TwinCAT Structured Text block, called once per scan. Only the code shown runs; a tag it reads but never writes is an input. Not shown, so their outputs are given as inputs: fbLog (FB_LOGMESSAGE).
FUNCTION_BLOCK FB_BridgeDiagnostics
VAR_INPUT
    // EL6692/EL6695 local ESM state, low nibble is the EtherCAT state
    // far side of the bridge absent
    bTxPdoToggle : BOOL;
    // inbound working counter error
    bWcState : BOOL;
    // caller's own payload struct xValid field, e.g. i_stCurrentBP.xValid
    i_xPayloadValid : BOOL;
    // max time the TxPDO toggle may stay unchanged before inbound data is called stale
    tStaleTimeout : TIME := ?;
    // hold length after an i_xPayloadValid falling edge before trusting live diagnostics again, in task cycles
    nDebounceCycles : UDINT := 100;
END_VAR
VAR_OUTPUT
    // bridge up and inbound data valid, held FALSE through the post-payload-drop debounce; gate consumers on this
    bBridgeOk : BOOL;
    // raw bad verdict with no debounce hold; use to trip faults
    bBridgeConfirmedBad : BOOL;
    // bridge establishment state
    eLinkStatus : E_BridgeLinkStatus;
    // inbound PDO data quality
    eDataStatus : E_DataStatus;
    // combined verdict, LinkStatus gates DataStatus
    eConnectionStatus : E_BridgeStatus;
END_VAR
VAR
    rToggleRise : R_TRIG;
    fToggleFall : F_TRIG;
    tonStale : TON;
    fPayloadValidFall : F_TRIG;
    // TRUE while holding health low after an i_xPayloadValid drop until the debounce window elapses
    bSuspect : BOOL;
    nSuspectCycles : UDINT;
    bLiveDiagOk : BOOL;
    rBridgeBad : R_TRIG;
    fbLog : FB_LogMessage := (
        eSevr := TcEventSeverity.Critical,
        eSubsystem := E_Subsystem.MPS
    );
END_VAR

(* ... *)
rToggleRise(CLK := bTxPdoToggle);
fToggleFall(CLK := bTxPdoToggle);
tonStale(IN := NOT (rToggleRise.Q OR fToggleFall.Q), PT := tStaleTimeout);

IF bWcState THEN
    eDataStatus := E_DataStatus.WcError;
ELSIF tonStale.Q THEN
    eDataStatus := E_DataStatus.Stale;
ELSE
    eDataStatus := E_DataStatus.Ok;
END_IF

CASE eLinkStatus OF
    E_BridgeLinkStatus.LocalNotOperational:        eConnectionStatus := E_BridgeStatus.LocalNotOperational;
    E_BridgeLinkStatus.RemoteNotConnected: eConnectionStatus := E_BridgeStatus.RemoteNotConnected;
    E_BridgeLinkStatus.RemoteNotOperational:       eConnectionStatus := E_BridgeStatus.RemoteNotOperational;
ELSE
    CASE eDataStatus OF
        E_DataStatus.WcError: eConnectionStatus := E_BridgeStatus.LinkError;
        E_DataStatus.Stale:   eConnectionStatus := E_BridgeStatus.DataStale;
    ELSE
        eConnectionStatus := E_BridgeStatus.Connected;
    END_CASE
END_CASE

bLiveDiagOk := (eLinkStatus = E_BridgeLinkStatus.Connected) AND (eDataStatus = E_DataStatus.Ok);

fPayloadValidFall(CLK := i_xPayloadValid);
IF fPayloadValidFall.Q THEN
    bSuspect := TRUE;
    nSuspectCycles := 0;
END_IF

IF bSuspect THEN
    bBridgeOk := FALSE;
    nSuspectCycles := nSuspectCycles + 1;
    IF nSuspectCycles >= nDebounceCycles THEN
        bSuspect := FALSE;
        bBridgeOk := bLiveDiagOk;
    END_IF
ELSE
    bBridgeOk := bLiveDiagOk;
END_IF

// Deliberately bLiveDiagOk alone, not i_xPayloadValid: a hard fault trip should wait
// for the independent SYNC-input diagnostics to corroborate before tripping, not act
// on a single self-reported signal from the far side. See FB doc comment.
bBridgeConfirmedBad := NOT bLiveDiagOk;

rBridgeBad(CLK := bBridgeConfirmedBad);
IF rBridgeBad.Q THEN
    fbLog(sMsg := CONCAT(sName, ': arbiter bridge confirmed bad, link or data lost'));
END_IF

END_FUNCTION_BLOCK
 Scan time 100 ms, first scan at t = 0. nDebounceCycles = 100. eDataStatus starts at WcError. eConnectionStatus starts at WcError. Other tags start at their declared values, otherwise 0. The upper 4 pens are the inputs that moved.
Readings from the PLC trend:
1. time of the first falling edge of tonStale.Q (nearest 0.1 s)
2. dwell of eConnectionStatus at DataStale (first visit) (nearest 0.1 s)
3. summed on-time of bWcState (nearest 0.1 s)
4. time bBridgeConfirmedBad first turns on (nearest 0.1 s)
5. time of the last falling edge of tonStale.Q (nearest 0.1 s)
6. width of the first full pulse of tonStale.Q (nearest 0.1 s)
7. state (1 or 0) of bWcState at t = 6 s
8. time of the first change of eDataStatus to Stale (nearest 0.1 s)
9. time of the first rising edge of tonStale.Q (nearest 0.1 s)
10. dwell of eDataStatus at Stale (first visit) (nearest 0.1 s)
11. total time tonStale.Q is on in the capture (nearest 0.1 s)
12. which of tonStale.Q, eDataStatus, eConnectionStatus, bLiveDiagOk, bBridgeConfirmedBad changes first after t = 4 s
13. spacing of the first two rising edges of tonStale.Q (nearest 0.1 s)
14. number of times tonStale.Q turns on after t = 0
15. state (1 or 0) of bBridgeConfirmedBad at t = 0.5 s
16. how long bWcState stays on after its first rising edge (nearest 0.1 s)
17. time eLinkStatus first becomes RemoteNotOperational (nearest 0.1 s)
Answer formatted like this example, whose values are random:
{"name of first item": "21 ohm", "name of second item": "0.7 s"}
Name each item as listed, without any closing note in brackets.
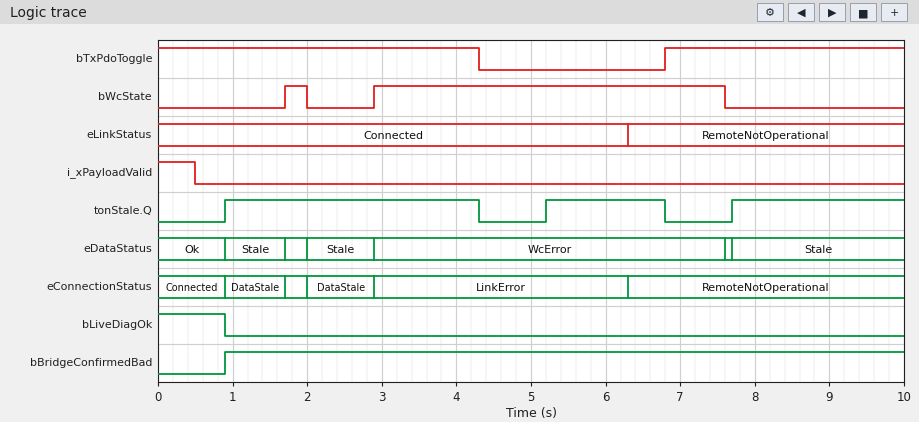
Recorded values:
{"time of the first falling edge of tonStale.Q": "4.3 s", "dwell of eConnectionStatus at DataStale (first visit)": "0.8 s", "summed on-time of bWcState": "5.0 s", "time bBridgeConfirmedBad first turns on": "0.9 s", "time of the last falling edge of tonStale.Q": "6.8 s", "width of the first full pulse of tonStale.Q": "3.4 s", "state (1 or 0) of bWcState at t = 6 s": "1", "time of the first change of eDataStatus to Stale": "0.9 s", "time of the first rising edge of tonStale.Q": "0.9 s", "dwell of eDataStatus at Stale (first visit)": "0.8 s", "total time tonStale.Q is on in the capture": "7.3 s", "which of tonStale.Q, eDataStatus, eConnectionStatus, bLiveDiagOk, bBridgeConfirmedBad changes first after t = 4 s": "tonStale.Q", "spacing of the first two rising edges of tonStale.Q": "4.3 s", "number of times tonStale.Q turns on after t = 0": "3", "state (1 or 0) of bBridgeConfirmedBad at t = 0.5 s": "0", "how long bWcState stays on after its first rising edge": "0.3 s", "time eLinkStatus first becomes RemoteNotOperational": "6.3 s"}
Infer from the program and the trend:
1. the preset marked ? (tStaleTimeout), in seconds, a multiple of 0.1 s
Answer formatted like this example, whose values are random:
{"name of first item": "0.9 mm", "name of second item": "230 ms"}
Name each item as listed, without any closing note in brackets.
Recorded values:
{"the preset marked ? (tStaleTimeout), in seconds, a multiple of 0.1 s": "0.8 s"}
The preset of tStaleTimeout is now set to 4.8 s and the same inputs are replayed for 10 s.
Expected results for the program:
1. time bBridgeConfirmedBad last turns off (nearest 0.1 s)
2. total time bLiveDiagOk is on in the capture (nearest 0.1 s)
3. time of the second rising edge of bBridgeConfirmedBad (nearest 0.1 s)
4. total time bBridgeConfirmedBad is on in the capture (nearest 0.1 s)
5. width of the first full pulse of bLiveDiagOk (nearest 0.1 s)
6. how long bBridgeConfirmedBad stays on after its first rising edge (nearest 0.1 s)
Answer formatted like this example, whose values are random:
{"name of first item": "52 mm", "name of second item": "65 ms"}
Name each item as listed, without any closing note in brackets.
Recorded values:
{"time bBridgeConfirmedBad last turns off": "2.0 s", "total time bLiveDiagOk is on in the capture": "2.6 s", "time of the second rising edge of bBridgeConfirmedBad": "2.9 s", "total time bBridgeConfirmedBad is on in the capture": "7.4 s", "width of the first full pulse of bLiveDiagOk": "0.9 s", "how long bBridgeConfirmedBad stays on after its first rising edge": "0.3 s"}
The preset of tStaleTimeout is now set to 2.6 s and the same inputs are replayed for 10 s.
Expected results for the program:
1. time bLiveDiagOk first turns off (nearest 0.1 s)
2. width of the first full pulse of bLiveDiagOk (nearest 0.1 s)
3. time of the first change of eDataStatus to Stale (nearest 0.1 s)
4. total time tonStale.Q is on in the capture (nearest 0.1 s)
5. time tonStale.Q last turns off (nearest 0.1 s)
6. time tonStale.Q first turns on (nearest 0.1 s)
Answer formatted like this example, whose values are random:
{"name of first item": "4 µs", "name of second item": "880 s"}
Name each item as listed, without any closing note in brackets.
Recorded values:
{"time bLiveDiagOk first turns off": "1.7 s", "width of the first full pulse of bLiveDiagOk": "0.7 s", "time of the first change of eDataStatus to Stale": "2.7 s", "total time tonStale.Q is on in the capture": "2.1 s", "time tonStale.Q last turns off": "4.3 s", "time tonStale.Q first turns on": "2.7 s"}
